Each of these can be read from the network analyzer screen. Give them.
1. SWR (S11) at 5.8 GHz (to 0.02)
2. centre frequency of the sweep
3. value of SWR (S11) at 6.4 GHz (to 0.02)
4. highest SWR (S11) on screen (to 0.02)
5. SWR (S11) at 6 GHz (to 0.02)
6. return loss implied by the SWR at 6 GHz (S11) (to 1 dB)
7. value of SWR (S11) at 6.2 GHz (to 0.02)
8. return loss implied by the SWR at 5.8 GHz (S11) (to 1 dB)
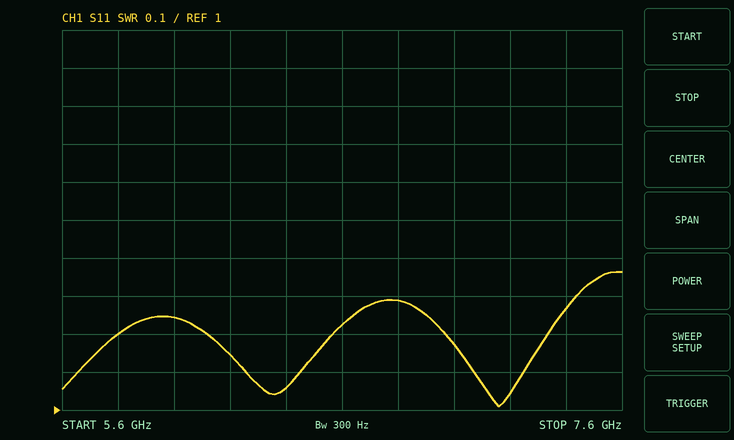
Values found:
1.20
6.6 GHz
1.06
1.36
1.24
19 dB
1.14
21 dB
